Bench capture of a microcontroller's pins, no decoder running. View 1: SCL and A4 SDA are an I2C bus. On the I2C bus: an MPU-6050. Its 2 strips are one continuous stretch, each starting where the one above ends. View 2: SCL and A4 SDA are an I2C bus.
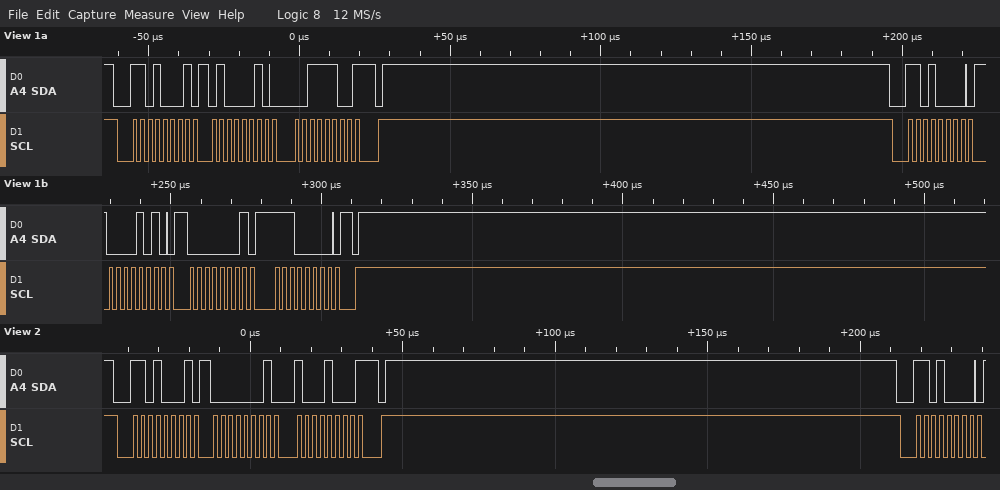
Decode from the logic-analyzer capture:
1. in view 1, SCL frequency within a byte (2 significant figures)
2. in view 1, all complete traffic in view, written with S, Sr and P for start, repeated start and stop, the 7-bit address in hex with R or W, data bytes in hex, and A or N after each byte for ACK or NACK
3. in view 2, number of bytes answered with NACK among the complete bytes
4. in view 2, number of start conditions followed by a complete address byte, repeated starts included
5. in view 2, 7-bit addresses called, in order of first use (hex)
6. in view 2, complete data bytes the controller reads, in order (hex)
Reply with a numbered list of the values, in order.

1. 400 kHz
2. S 68R A 42 A 3C N P S 68W A 0A A 01 A E0 A P
3. 1
4. 2
5. 0x68
6. 01 88
